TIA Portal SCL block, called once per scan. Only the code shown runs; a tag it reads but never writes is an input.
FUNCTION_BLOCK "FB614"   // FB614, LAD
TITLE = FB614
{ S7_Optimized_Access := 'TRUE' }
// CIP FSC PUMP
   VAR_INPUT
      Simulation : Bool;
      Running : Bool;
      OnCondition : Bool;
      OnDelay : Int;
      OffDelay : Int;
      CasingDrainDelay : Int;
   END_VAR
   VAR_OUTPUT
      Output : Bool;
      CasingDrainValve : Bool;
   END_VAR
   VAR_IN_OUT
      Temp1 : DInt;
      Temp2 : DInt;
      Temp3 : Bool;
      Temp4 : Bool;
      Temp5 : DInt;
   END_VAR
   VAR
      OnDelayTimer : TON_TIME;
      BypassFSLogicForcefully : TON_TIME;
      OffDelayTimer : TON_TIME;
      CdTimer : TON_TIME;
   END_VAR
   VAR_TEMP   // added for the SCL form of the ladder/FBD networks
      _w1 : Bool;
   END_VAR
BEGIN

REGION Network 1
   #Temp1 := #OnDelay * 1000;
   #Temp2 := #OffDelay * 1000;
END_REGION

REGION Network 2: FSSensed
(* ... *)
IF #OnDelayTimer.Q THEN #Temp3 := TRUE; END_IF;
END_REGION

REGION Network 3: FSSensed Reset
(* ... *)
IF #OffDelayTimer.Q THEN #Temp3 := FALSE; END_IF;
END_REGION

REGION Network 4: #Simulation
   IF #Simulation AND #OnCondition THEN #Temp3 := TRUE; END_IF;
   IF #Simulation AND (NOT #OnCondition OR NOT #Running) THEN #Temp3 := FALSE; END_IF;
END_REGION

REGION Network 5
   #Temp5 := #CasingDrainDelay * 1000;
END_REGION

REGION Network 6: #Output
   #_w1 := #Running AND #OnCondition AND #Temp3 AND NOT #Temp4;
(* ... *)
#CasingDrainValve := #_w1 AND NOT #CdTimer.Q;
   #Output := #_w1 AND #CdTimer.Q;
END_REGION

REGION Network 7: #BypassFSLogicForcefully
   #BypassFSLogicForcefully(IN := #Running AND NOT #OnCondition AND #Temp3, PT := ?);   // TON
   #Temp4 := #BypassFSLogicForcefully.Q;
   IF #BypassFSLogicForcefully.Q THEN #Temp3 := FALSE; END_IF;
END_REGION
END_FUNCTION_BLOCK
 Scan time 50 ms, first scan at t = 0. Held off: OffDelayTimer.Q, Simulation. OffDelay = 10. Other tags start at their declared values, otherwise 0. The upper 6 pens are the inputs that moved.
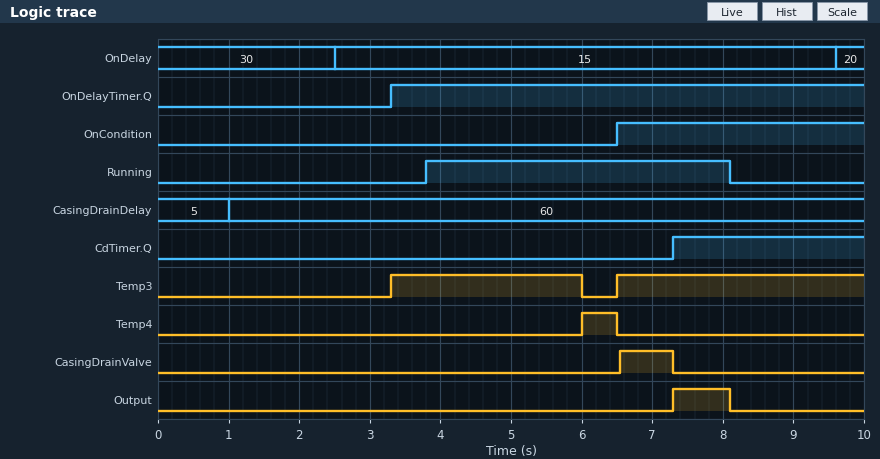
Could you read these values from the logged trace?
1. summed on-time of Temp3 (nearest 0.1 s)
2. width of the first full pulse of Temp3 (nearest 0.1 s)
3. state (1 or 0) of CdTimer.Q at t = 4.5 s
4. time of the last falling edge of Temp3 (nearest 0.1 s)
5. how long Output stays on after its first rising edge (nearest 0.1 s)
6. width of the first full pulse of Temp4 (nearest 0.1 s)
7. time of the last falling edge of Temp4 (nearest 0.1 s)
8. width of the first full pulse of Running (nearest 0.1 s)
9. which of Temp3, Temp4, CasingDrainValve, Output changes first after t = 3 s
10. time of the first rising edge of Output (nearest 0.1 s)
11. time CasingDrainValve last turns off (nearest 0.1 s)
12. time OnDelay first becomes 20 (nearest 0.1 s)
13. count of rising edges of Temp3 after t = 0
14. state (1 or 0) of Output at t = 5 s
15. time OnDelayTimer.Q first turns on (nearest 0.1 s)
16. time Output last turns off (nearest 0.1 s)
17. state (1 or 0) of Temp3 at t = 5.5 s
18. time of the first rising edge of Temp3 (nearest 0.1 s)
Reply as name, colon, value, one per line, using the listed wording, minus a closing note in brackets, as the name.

summed on-time of Temp3: 6.2 s
width of the first full pulse of Temp3: 2.7 s
state (1 or 0) of CdTimer.Q at t = 4.5 s: 0
time of the last falling edge of Temp3: 6.0 s
how long Output stays on after its first rising edge: 0.8 s
width of the first full pulse of Temp4: 0.5 s
time of the last falling edge of Temp4: 6.5 s
width of the first full pulse of Running: 4.3 s
which of Temp3, Temp4, CasingDrainValve, Output changes first after t = 3 s: Temp3
time of the first rising edge of Output: 7.3 s
time CasingDrainValve last turns off: 7.3 s
time OnDelay first becomes 20: 9.6 s
count of rising edges of Temp3 after t = 0: 2
state (1 or 0) of Output at t = 5 s: 0
time OnDelayTimer.Q first turns on: 3.3 s
time Output last turns off: 8.1 s
state (1 or 0) of Temp3 at t = 5.5 s: 1
time of the first rising edge of Temp3: 3.3 s
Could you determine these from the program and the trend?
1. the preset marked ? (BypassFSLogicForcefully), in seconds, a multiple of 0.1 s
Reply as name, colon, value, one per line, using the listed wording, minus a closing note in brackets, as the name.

the preset marked ? (BypassFSLogicForcefully), in seconds, a multiple of 0.1 s: 2.2 s
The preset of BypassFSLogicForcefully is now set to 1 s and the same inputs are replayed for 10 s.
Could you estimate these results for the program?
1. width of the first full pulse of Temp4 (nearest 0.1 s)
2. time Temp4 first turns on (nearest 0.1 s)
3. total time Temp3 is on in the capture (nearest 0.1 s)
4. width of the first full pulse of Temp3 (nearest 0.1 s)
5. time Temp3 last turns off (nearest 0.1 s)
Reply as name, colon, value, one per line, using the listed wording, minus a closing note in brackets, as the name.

width of the first full pulse of Temp4: 1.7 s
time Temp4 first turns on: 4.8 s
total time Temp3 is on in the capture: 5.0 s
width of the first full pulse of Temp3: 1.5 s
time Temp3 last turns off: 4.8 s
